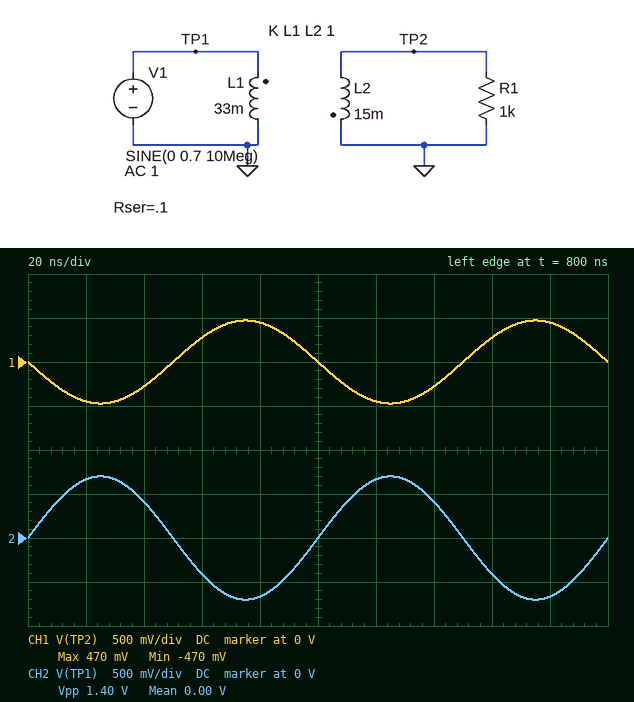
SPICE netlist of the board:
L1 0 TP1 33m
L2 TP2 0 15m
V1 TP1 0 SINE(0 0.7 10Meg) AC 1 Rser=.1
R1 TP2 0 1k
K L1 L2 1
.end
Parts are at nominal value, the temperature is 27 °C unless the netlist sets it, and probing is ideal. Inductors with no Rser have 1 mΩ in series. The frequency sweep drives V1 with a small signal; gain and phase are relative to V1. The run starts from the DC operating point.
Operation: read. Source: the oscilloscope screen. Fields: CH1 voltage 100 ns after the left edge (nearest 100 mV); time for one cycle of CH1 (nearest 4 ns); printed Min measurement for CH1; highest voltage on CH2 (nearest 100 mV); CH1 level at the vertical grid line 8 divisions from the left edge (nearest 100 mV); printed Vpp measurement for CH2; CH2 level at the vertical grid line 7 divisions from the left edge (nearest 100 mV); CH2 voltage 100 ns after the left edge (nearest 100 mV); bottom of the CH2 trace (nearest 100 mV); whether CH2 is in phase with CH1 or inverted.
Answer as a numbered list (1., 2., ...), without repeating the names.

1. 0 V
2. 100 ns
3. -470 mV
4. 700 mV
5. 300 mV
6. 1.40 V
7. 400 mV
8. 0 V
9. -700 mV
10. inverted
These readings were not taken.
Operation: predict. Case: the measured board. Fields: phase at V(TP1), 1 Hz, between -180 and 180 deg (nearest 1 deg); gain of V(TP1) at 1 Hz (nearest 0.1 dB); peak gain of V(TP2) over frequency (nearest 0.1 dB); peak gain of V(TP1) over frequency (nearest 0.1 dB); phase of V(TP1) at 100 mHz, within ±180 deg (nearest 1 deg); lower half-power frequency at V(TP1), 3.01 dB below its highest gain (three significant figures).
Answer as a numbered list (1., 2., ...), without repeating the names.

1. 26 deg
2. -0.9 dB
3. -3.4 dB
4. 0 dB
5. 76 deg
6. 487 mHz
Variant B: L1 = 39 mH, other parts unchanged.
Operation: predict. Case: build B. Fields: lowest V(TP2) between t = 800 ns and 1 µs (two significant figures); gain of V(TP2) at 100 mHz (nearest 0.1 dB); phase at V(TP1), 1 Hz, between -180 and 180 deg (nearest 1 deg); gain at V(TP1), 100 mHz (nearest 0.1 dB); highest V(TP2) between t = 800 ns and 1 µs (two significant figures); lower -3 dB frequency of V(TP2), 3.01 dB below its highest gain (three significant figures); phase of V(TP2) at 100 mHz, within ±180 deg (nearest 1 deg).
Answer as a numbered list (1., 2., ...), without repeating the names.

1. -430 mV
2. -16.7 dB
3. 22 deg
4. -12.5 dB
5. 430 mV
6. 412 mHz
7. -104 deg
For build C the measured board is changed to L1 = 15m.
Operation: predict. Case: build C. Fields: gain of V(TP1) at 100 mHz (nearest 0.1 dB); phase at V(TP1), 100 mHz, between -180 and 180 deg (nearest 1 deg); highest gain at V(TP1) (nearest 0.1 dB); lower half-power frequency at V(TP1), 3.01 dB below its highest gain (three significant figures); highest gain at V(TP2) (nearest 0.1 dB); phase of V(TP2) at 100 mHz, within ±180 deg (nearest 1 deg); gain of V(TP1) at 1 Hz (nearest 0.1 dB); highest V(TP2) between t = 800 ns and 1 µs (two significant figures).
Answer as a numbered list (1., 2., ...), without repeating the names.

1. -20.6 dB
2. 79 deg
3. 0 dB
4. 1.07 Hz
5. 0 dB
6. -95 deg
7. -3.3 dB
8. 700 mV
